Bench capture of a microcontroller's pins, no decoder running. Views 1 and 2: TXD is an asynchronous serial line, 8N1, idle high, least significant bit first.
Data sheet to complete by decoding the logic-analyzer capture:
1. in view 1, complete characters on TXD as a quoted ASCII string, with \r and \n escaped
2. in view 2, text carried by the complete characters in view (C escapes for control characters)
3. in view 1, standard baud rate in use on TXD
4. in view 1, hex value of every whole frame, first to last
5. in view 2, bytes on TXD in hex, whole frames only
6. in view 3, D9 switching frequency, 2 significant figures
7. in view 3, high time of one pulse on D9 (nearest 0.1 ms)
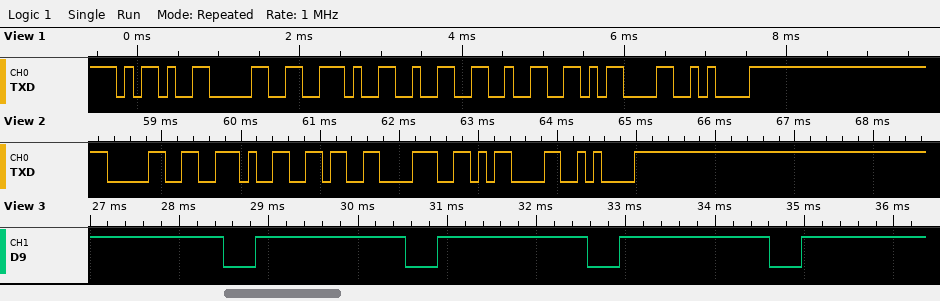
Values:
"-0.22\r\n"
"0.68\r\n"
9600 baud
2D 30 2E 32 32 0D 0A
30 2E 36 38 0D 0A
490 Hz
1.7 ms
